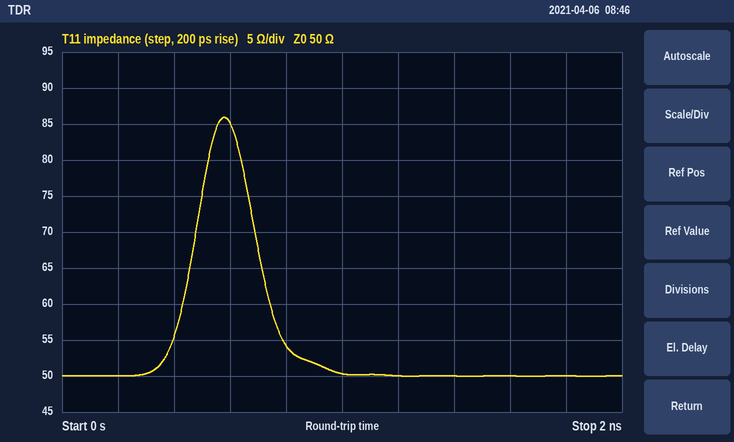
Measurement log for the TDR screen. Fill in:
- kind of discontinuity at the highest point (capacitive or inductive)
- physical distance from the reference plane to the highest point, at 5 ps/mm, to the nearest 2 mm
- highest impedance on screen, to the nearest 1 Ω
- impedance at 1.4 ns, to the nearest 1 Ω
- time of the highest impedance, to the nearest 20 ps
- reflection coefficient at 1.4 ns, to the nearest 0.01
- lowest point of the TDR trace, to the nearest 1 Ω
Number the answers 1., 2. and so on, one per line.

1. inductive
2. 58 mm
3. 86 Ω
4. 50 Ω
5. 580 ps
6. 0.00
7. 50 Ω
